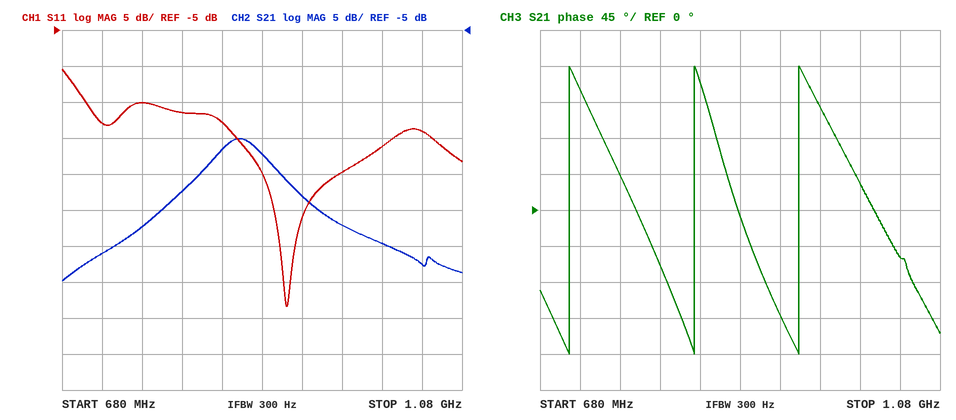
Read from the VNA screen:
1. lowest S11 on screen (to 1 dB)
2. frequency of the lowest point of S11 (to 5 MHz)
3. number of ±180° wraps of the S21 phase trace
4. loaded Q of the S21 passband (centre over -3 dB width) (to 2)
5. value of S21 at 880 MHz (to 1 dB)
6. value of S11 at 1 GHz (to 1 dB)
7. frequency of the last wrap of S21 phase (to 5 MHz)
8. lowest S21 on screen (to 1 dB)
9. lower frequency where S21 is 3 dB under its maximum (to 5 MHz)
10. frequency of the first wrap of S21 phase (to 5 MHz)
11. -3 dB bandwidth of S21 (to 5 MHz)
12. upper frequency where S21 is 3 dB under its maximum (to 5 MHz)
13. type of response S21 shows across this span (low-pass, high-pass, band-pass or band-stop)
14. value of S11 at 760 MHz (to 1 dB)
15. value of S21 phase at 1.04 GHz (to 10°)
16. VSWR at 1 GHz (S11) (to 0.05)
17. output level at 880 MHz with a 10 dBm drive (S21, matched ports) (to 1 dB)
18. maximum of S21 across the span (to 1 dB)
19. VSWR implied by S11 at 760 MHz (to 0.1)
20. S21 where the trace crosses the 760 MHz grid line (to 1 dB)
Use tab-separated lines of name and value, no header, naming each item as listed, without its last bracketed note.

lowest S11 on screen	-43 dB
frequency of the lowest point of S11	905 MHz
number of ±180° wraps of the S21 phase trace	3
loaded Q of the S21 passband (centre over -3 dB width)	16
value of S21 at 880 MHz	-22 dB
value of S11 at 1 GHz	-21 dB
frequency of the last wrap of S21 phase	940 MHz
lowest S21 on screen	-40 dB
lower frequency where S21 is 3 dB under its maximum	830 MHz
frequency of the first wrap of S21 phase	710 MHz
-3 dB bandwidth of S21	55 MHz
upper frequency where S21 is 3 dB under its maximum	885 MHz
type of response S21 shows across this span	band-pass
value of S11 at 760 MHz	-15 dB
value of S21 phase at 1.04 GHz	-60°
VSWR at 1 GHz (S11)	1.20
output level at 880 MHz with a 10 dBm drive (S21, matched ports)	-12 dBm
maximum of S21 across the span	-20 dB
VSWR implied by S11 at 760 MHz	1.4
S21 where the trace crosses the 760 MHz grid line	-32 dB
